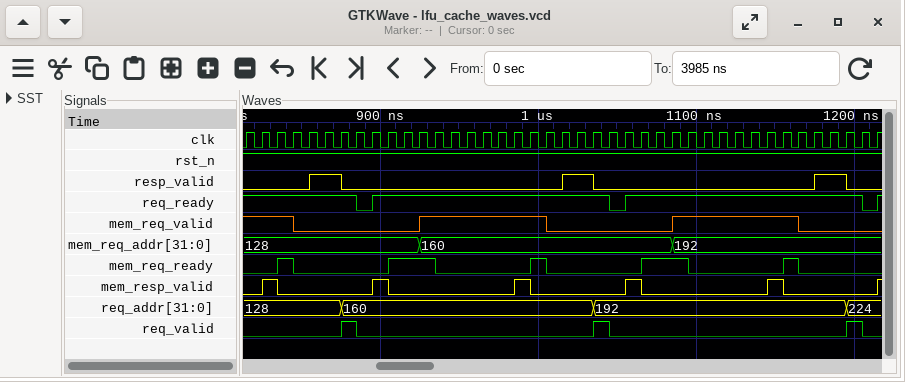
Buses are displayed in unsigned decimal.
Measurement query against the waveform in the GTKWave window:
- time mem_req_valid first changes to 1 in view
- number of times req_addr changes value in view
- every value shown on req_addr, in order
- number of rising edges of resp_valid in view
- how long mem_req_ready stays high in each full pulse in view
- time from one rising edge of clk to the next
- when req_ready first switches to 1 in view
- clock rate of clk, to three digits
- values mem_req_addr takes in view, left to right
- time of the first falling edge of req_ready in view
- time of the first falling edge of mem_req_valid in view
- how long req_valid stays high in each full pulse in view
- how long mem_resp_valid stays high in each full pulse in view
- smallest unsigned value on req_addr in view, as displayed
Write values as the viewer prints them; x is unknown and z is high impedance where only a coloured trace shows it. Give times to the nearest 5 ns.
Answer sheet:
925 ns
3
128, 160, 192, 224
3
10 ns, 30 ns, 10 ns, 30 ns, 10 ns
10 ns
895 ns
100 MHz
128, 160, 192
885 ns
845 ns
10 ns, 10 ns, 10 ns
10 ns, 10 ns, 10 ns, 10 ns, 10 ns
128
